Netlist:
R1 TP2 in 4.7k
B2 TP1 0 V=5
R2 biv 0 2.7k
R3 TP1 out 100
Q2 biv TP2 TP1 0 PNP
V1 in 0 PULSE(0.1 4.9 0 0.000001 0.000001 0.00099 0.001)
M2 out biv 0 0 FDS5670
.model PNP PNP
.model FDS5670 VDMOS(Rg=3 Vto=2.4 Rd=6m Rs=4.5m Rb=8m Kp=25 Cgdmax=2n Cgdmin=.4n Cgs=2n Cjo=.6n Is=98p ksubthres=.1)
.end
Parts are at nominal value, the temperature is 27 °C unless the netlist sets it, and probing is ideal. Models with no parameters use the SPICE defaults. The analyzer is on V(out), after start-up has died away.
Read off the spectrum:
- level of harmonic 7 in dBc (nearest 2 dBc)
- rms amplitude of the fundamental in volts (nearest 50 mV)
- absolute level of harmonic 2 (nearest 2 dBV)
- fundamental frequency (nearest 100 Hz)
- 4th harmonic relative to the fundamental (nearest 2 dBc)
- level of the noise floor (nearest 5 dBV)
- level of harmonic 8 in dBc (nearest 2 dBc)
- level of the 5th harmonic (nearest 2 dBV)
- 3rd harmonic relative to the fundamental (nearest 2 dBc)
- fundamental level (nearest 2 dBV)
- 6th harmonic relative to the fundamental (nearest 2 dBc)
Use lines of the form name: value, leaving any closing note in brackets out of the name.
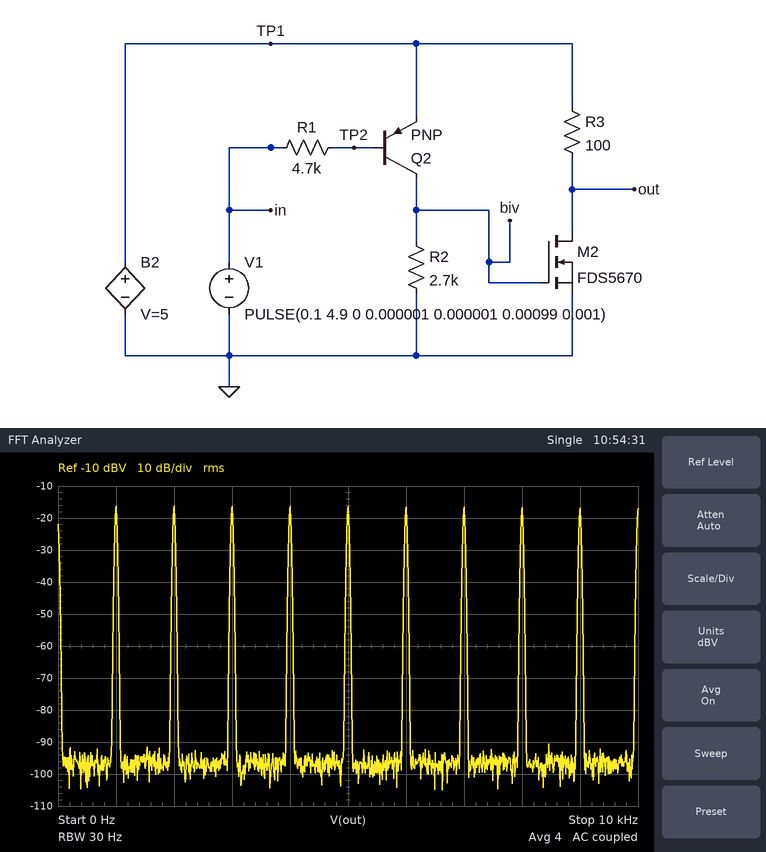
level of harmonic 7 in dBc: 0 dBc
rms amplitude of the fundamental in volts: 150 mV
absolute level of harmonic 2: -16 dBV
fundamental frequency: 1.0 kHz
4th harmonic relative to the fundamental: 0 dBc
level of the noise floor: -95 dBV
level of harmonic 8 in dBc: 0 dBc
level of the 5th harmonic: -16 dBV
3rd harmonic relative to the fundamental: 0 dBc
fundamental level: -16 dBV
6th harmonic relative to the fundamental: 0 dBc
